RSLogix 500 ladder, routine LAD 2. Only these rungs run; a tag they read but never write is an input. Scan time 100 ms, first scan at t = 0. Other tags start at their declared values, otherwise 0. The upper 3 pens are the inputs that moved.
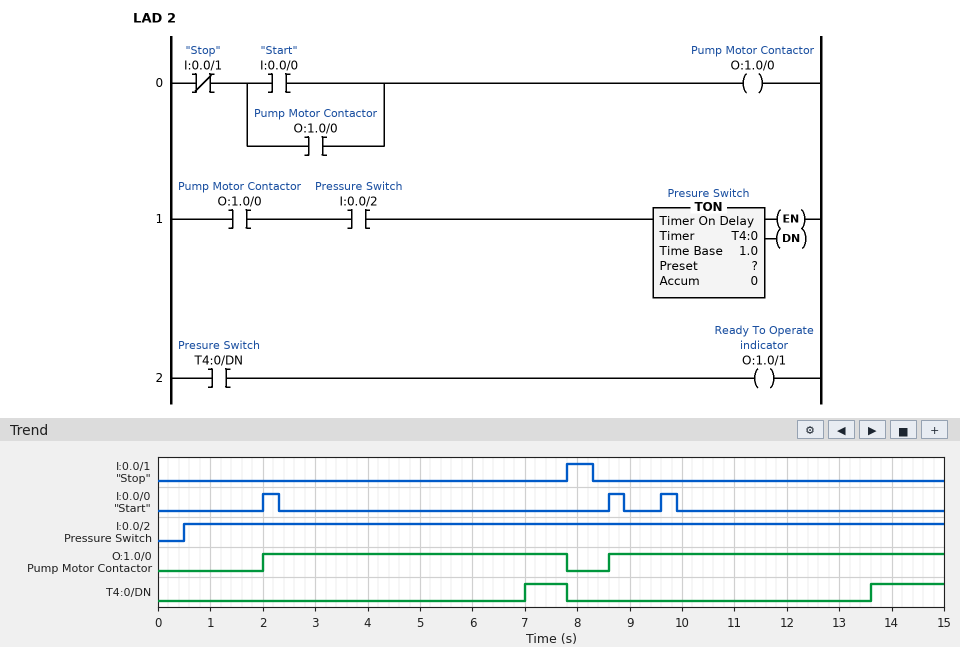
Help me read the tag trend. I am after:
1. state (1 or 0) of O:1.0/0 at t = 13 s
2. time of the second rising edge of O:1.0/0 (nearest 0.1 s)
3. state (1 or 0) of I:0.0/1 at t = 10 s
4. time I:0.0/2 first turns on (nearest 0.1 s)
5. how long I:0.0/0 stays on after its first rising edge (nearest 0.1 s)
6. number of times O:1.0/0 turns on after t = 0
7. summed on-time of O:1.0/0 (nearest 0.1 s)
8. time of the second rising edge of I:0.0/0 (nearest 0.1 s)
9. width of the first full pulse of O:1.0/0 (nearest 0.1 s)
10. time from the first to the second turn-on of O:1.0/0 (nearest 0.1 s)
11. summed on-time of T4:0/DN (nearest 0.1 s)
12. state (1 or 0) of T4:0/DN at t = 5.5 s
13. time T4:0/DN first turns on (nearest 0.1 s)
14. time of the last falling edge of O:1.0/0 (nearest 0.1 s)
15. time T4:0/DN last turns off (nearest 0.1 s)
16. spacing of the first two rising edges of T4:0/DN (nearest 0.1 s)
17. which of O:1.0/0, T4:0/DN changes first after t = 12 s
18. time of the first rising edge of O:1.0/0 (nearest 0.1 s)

1
8.6 s
0
0.5 s
0.3 s
2
12.2 s
8.6 s
5.8 s
6.6 s
2.2 s
0
7.0 s
7.8 s
7.8 s
6.6 s
T4:0/DN
2.0 s
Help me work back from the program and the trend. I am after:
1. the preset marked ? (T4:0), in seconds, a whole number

5 s
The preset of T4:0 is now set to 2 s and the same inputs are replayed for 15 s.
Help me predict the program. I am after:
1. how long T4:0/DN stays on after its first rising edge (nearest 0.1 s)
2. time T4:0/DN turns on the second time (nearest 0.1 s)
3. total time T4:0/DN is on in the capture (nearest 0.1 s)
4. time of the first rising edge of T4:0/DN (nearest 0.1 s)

3.8 s
10.6 s
8.2 s
4.0 s
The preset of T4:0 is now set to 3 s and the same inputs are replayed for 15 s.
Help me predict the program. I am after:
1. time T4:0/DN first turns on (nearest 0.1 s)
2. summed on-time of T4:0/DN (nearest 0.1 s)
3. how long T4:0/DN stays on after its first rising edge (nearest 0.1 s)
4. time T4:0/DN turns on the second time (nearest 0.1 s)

5.0 s
6.2 s
2.8 s
11.6 s
